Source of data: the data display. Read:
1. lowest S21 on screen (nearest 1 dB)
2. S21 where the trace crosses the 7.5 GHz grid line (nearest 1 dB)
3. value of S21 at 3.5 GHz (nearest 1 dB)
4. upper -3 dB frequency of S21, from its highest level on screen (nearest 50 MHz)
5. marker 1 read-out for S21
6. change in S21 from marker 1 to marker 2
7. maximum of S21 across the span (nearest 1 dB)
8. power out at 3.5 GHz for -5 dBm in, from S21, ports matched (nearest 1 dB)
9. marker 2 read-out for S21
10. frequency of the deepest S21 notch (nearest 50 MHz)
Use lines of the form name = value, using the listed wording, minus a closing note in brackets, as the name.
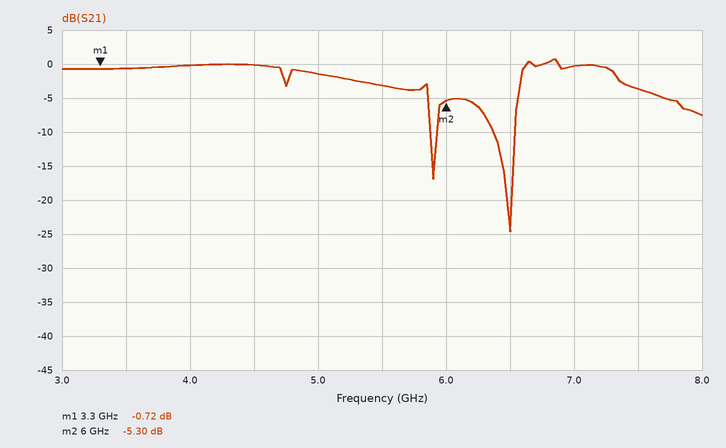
lowest S21 on screen = -25 dB
S21 where the trace crosses the 7.5 GHz grid line = -4 dB
value of S21 at 3.5 GHz = -1 dB
upper -3 dB frequency of S21, from its highest level on screen = 7.35 GHz
marker 1 read-out for S21 = -0.72 dB
change in S21 from marker 1 to marker 2 = -4.58 dB
maximum of S21 across the span = 1 dB
power out at 3.5 GHz for -5 dBm in, from S21, ports matched = -6 dBm
marker 2 read-out for S21 = -5.30 dB
frequency of the deepest S21 notch = 6.50 GHz
